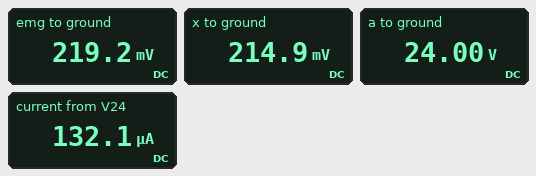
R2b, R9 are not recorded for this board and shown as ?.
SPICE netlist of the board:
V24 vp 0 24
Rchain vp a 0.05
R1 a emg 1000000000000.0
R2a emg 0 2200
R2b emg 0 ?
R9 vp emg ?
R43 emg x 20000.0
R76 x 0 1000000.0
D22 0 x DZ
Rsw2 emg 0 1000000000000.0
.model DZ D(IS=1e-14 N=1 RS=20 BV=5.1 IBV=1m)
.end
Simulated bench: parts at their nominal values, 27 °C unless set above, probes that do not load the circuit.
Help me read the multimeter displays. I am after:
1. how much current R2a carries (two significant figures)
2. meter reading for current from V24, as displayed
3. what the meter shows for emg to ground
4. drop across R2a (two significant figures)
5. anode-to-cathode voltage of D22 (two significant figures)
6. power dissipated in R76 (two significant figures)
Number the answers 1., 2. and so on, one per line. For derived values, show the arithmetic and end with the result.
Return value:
1. (219.2 mV) / 2.2 kΩ = 100 µA
2. 132.1 µA
3. 219.2 mV
4. 219.2 mV = 220 mV
5. 0 V - 214.9 mV = -210 mV
6. (214.9 mV)^2 / 1 MΩ = 46 nW
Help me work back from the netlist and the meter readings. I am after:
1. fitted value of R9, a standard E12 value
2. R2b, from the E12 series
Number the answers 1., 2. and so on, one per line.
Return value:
1. 180 kΩ
2. 6.8 kΩ
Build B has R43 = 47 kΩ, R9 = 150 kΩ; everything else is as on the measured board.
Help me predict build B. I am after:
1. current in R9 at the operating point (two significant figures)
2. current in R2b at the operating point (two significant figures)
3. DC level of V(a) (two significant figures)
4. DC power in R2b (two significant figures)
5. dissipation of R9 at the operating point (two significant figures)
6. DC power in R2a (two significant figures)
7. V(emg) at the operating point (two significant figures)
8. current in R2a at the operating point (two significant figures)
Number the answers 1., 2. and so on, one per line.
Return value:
1. 160 µA
2. 39 µA
3. 24 V
4. 10 µW
5. 3.8 mW
6. 31 µW
7. 260 mV
8. 120 µA
